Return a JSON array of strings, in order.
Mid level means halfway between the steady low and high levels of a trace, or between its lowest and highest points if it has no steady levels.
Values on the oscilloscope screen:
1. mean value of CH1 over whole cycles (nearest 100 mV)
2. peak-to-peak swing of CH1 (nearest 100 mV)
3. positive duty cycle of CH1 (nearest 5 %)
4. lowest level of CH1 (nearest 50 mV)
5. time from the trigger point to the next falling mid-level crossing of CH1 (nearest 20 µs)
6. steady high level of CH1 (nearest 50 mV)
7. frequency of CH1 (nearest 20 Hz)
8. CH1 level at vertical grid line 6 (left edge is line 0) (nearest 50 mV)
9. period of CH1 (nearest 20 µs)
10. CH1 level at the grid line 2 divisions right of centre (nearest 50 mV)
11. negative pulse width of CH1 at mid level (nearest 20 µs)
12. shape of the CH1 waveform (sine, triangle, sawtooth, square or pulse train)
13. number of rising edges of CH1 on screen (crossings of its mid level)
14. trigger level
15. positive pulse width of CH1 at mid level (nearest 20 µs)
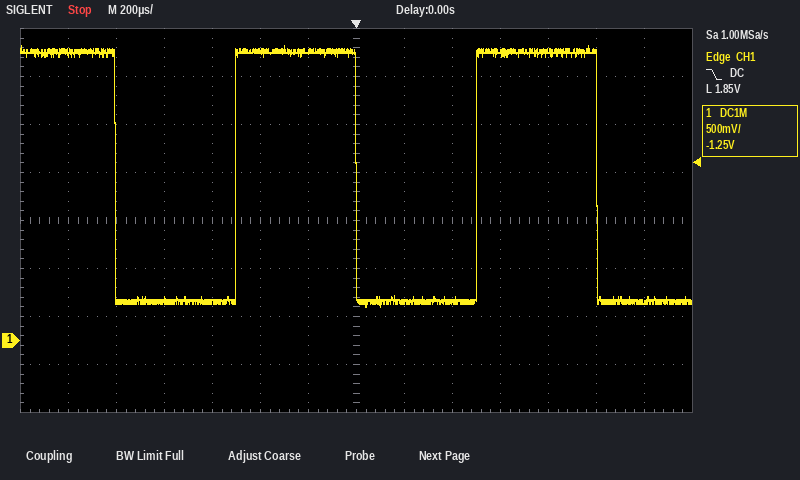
["1.7 V", "2.70 V", "50 %", "350 mV", "1.00 ms", "3.00 V", "1.00 kHz", "3.00 V", "1.00 ms", "400 mV", "500 µs", "square", "2", "1.85 V", "500 µs"]
